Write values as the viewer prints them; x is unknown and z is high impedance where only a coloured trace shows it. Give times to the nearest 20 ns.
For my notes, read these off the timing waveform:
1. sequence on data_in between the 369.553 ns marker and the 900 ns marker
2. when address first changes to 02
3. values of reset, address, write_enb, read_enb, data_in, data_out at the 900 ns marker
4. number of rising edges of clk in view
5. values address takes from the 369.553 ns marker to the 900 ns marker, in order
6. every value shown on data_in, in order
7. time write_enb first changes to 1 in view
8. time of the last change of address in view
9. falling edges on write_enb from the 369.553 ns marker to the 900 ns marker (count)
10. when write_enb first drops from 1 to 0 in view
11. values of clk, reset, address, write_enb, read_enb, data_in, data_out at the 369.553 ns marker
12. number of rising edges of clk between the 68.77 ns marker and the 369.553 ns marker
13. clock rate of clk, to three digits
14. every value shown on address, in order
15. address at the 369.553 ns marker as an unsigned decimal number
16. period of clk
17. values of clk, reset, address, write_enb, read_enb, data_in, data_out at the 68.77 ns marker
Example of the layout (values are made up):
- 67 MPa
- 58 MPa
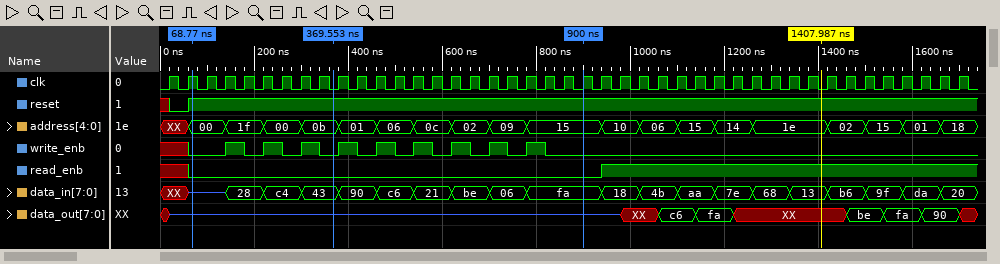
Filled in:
- 43, 90, c6, 21, be, 06, fa
- 620 ns
- reset=1, address=15, write_enb=0, read_enb=0, data_in=fa, data_out=z
- 43
- 0b, 01, 06, 0c, 02, 09, 15
- XX, z, 28, c4, 43, 90, c6, 21, be, 06, fa, 18, 4b, aa, 7e, 68, 13, b6, 9f, da, 20
- 140 ns
- 1660 ns
- 6
- 180 ns
- clk=0, reset=1, address=0b, write_enb=0, read_enb=0, data_in=43, data_out=z
- 7
- 25.0 MHz
- XX, 00, 1f, 00, 0b, 01, 06, 0c, 02, 09, 15, 10, 06, 15, 14, 1e, 02, 15, 01, 18
- 11
- 40 ns
- clk=1, reset=1, address=00, write_enb=0, read_enb=0, data_in=z, data_out=z
